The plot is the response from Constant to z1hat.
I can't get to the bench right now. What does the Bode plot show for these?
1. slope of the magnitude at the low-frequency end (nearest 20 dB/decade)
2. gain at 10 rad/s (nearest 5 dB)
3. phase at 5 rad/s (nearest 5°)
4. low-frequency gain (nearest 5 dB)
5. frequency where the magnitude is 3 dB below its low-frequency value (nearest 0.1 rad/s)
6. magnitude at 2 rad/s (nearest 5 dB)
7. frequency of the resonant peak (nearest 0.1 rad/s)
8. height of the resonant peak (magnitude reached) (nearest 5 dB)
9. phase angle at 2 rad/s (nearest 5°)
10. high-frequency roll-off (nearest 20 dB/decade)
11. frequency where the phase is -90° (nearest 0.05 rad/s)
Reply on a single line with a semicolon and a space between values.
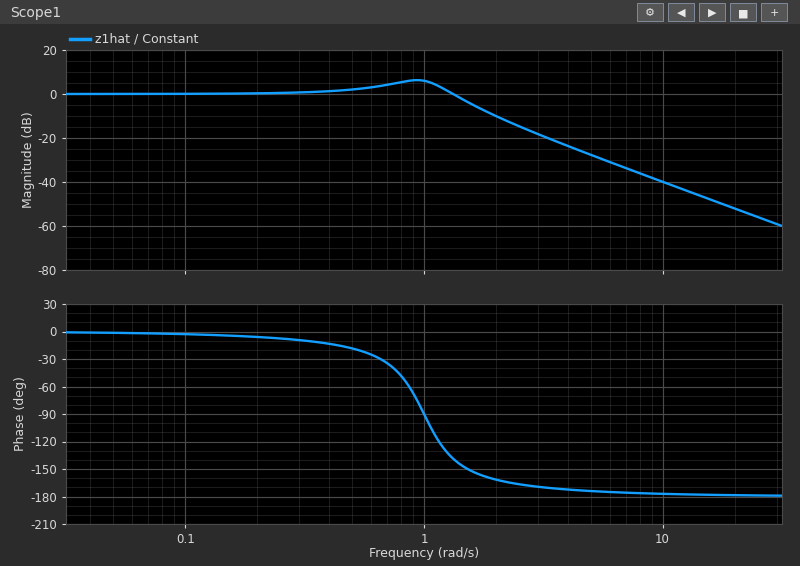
0 dB/decade; -40 dB; -175°; 0 dB; 1.5 rad/s; -10 dB; 0.9 rad/s; 5 dB; -160°; -40 dB/decade; 1.00 rad/s
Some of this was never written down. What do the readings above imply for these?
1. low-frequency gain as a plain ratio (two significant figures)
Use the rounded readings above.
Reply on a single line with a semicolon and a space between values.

1.0
